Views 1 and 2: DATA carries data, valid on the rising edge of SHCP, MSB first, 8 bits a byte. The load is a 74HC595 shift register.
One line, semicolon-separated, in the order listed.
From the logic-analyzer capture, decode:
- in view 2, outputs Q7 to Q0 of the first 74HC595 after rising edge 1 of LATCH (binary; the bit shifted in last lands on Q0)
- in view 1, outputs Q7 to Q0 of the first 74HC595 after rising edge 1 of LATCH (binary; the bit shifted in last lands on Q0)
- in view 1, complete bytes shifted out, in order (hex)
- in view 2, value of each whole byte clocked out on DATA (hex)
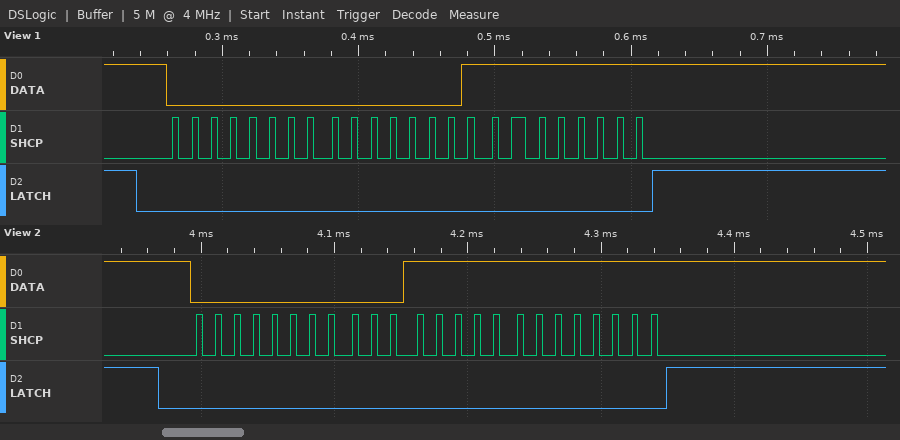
11111111; 11111111; 00 01 FF; 0x00 0x1F 0xFF
